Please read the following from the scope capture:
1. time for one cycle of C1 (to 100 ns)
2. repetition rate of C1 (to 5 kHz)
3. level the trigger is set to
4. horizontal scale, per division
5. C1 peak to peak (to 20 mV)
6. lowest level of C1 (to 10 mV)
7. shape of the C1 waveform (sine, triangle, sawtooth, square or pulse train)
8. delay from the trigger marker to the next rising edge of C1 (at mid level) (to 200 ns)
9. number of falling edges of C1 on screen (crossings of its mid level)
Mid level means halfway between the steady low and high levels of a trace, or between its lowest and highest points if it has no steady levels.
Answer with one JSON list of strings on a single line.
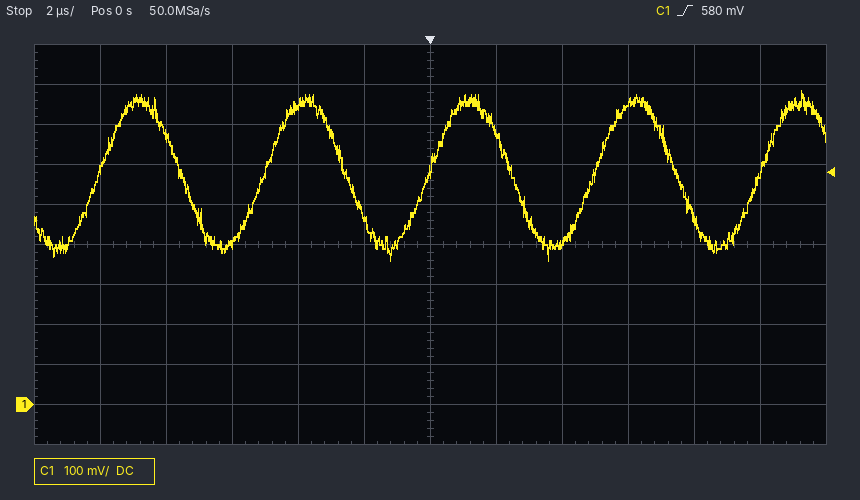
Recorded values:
["5.0 µs", "200 kHz", "580 mV", "2 µs", "420 mV", "360 mV", "sine", "5.0 µs", "4"]
